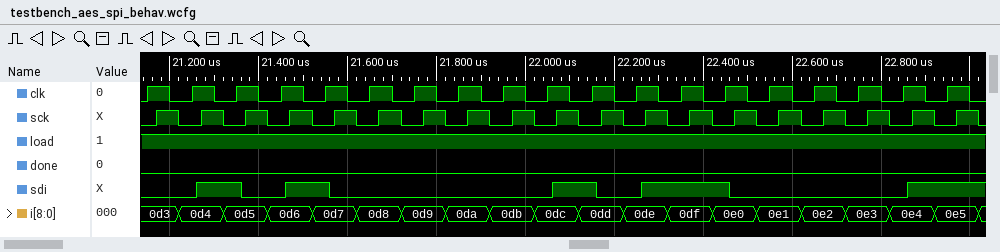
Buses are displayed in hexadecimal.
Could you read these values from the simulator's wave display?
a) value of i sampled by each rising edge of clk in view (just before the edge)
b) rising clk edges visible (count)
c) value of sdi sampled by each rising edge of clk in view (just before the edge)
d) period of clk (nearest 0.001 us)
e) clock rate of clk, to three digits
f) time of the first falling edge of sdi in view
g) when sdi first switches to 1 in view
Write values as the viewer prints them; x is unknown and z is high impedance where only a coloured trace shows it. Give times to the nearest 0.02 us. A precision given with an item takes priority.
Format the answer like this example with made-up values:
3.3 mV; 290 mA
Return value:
0d3, 0d4, 0d5, 0d6, 0d7, 0d8, 0d9, 0da, 0db, 0dc, 0dd, 0de, 0df, 0e0, 0e1, 0e2, 0e3, 0e4, 0e5; 19; 0 0 1 0 1 0 0 0 0 0 1 0 1 1 0 0 0 0 1; 0.1 us; 10.0 MHz; 21.36 us; 21.26 us
